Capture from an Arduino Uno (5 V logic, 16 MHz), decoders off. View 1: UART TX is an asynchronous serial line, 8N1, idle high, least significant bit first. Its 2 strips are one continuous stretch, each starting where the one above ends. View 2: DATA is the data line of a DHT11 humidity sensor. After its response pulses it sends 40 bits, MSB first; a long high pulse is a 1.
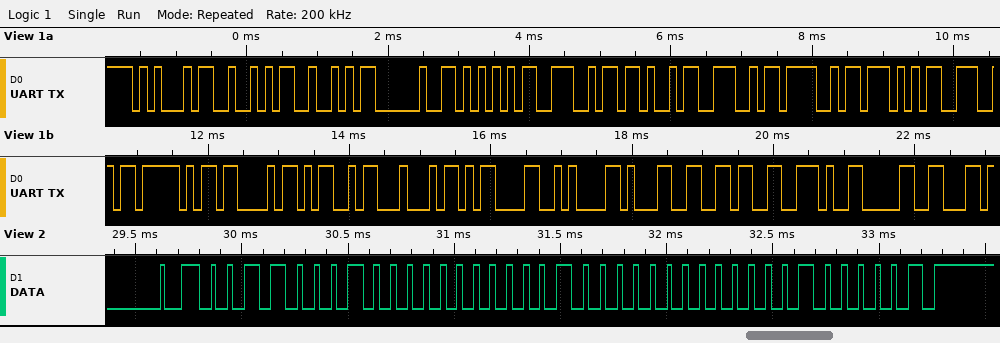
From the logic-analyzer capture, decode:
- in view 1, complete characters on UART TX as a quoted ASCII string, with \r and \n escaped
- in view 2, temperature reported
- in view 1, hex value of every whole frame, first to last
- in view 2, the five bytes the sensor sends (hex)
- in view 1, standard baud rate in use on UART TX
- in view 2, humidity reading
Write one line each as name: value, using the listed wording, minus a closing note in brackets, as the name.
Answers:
in view 1, complete characters on UART TX as a quoted ASCII string, with \r and \n escaped: "ERR UNKNOWN_CMD\r\n16.0"
in view 2, temperature reported: 16.0 °C
in view 1, hex value of every whole frame, first to last: 0x45 0x52 0x52 0x20 0x55 0x4E 0x4B 0x4E 0x4F 0x57 0x4E 0x5F 0x43 0x4D 0x44 0x0D 0x0A 0x31 0x36 0x2E 0x30
in view 2, the five bytes the sensor sends: 31 00 10 00 41
in view 1, standard baud rate in use on UART TX: 9600 baud
in view 2, humidity reading: 49 %
